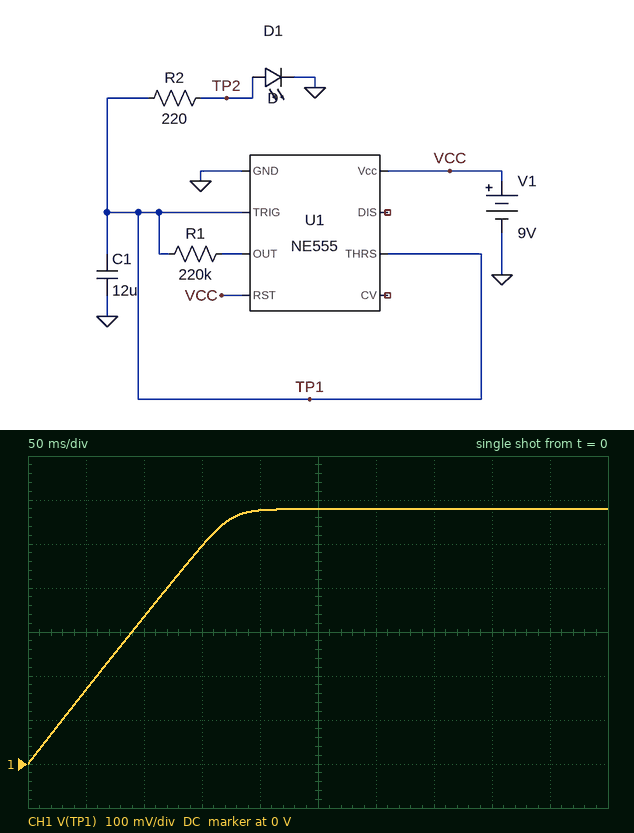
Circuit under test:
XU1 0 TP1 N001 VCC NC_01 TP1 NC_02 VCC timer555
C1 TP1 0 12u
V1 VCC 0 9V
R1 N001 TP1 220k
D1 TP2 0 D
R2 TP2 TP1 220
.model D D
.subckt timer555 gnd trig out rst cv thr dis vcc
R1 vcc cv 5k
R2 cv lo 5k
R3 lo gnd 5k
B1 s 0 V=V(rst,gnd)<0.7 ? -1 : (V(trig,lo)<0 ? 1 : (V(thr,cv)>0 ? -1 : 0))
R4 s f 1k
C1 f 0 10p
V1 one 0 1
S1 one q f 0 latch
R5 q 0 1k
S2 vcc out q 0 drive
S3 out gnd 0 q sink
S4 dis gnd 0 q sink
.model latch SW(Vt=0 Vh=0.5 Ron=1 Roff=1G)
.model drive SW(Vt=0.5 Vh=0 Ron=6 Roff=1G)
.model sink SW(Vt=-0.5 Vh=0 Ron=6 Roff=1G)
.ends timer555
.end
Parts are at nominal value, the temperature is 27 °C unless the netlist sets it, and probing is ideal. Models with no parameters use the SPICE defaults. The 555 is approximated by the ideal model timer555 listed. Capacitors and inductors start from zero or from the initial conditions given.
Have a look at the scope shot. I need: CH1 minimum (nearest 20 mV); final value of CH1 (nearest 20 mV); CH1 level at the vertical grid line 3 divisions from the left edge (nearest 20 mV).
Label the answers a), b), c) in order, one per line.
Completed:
a) 0 V
b) 580 mV
c) 500 mV
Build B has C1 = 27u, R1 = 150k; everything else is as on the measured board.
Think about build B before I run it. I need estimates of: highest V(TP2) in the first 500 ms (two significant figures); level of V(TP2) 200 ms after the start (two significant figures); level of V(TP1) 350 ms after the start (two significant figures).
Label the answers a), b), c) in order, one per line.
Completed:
a) 580 mV
b) 430 mV
c) 590 mV
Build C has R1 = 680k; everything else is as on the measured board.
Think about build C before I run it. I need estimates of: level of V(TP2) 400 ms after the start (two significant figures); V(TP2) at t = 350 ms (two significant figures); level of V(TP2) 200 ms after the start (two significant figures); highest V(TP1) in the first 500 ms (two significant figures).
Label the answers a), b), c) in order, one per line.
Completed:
a) 430 mV
b) 380 mV
c) 220 mV
d) 520 mV
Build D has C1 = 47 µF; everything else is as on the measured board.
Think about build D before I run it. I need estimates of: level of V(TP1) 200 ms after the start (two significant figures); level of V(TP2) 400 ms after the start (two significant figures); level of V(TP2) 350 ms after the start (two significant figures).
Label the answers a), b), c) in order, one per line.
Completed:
a) 170 mV
b) 340 mV
c) 300 mV
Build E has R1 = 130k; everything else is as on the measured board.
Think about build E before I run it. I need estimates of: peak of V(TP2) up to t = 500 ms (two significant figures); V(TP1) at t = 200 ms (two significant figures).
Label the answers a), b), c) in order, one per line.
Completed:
a) 580 mV
b) 600 mV
